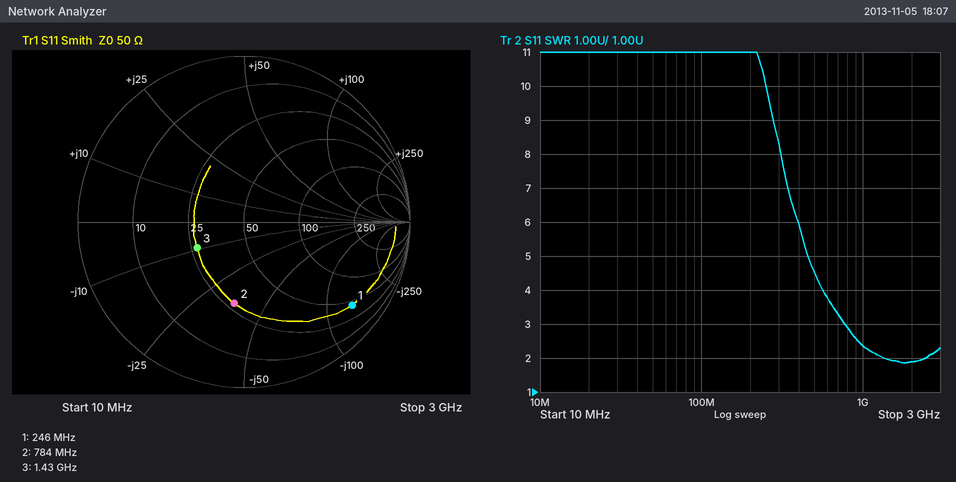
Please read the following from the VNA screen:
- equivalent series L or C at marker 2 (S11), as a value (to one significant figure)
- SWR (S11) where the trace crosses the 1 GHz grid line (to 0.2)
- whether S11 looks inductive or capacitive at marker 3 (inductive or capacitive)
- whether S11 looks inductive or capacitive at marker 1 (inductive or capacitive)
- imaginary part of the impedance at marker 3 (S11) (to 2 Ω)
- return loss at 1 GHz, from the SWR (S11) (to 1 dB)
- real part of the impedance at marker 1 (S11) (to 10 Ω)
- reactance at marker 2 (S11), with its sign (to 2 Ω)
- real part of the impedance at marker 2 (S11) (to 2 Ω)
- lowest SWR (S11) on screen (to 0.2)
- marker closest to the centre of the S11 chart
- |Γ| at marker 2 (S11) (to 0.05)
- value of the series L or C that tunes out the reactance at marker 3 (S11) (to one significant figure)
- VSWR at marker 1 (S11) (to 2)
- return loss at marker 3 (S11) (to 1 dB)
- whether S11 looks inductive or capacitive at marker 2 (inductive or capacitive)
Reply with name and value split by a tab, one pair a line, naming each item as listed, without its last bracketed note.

equivalent series L or C at marker 2 (S11), as a value	6 pF
SWR (S11) where the trace crosses the 1 GHz grid line	2.4
whether S11 looks inductive or capacitive at marker 3	capacitive
whether S11 looks inductive or capacitive at marker 1	capacitive
imaginary part of the impedance at marker 3 (S11)	-10 Ω
return loss at 1 GHz, from the SWR (S11)	8 dB
real part of the impedance at marker 1 (S11)	40 Ω
reactance at marker 2 (S11), with its sign	-36 Ω
real part of the impedance at marker 2 (S11)	28 Ω
lowest SWR (S11) on screen	1.8
marker closest to the centre of the S11 chart	marker 3
|Γ| at marker 2 (S11)	0.50
value of the series L or C that tunes out the reactance at marker 3 (S11)	1 nH
VSWR at marker 1 (S11)	10
return loss at marker 3 (S11)	10 dB
whether S11 looks inductive or capacitive at marker 2	capacitive
